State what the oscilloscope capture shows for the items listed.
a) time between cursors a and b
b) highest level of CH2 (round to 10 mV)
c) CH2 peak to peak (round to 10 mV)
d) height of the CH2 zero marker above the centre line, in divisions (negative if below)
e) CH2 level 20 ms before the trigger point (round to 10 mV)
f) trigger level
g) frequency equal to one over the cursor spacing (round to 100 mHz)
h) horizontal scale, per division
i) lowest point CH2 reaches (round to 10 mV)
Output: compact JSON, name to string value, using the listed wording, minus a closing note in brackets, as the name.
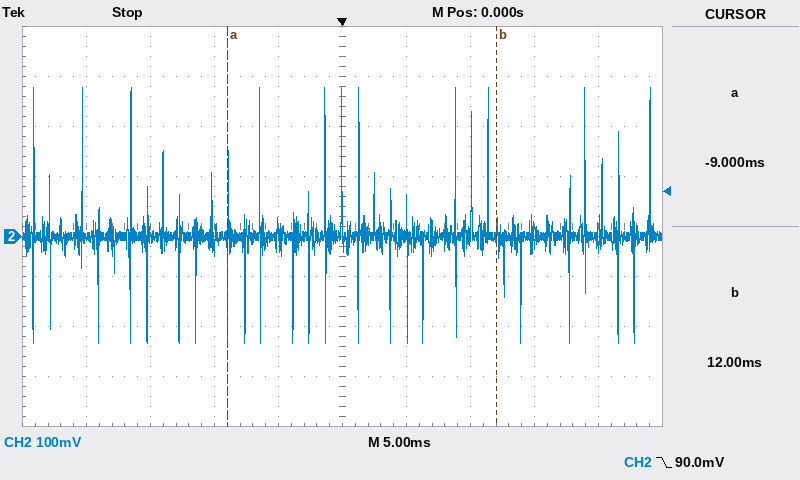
{"time between cursors a and b": "21.0 ms", "highest level of CH2": "300 mV", "CH2 peak to peak": "510 mV", "height of the CH2 zero marker above the centre line, in divisions": "-0.2 div", "CH2 level 20 ms before the trigger point": "0 mV", "trigger level": "90.0 mV", "frequency equal to one over the cursor spacing": "47.6 Hz", "horizontal scale, per division": "5 ms", "lowest point CH2 reaches": "-210 mV"}
